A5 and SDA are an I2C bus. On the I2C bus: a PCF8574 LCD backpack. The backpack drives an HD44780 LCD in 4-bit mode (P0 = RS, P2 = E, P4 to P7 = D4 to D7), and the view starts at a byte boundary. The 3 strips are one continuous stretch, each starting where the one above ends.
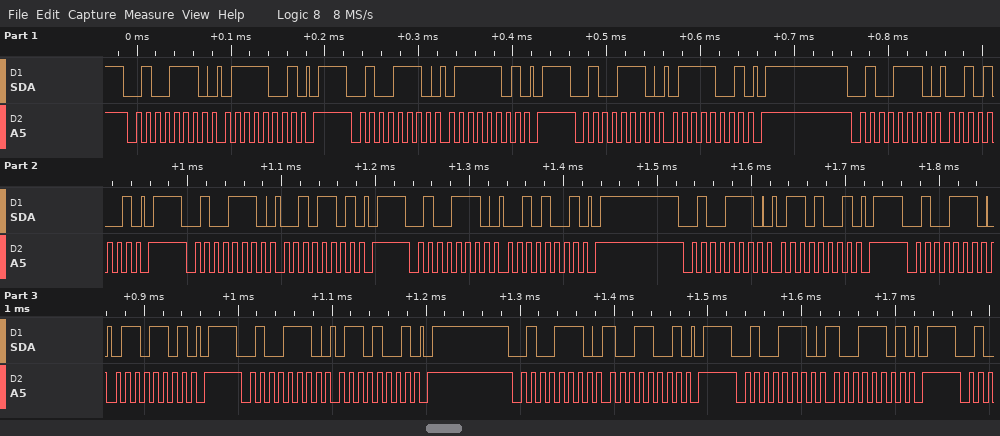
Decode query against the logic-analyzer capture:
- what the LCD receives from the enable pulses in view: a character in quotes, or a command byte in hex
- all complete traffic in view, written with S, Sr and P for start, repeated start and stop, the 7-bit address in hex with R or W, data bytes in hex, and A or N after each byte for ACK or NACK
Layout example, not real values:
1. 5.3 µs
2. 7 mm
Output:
1. 'r'
2. S 27W A 79 A P S 27W A 7D A P S 27W A 79 A P S 27W A 29 A P S 27W A 2D A P S 27W A 29 A P S 27W A 69 A P S 27W A 6D A P S 27W A 69 A P S 27W A 99 A P S 27W A 9D A P
